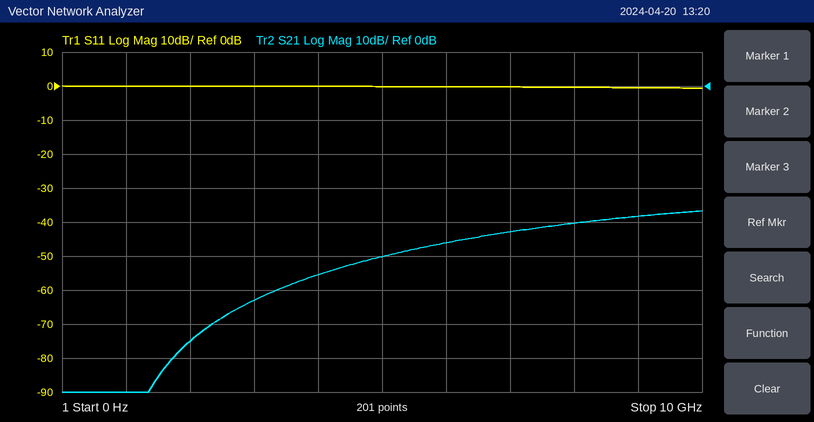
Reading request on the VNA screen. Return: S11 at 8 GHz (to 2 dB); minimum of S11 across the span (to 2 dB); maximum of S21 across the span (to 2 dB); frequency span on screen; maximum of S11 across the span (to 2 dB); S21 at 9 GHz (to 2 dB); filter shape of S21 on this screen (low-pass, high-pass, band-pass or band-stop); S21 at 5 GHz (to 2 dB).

0 dB
0 dB
-36 dB
10 GHz
0 dB
-38 dB
high-pass
-50 dB
